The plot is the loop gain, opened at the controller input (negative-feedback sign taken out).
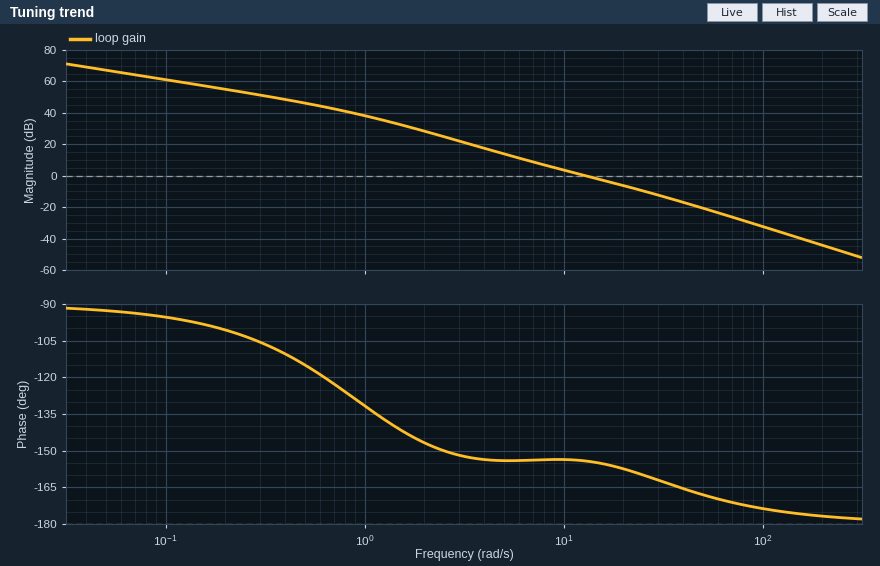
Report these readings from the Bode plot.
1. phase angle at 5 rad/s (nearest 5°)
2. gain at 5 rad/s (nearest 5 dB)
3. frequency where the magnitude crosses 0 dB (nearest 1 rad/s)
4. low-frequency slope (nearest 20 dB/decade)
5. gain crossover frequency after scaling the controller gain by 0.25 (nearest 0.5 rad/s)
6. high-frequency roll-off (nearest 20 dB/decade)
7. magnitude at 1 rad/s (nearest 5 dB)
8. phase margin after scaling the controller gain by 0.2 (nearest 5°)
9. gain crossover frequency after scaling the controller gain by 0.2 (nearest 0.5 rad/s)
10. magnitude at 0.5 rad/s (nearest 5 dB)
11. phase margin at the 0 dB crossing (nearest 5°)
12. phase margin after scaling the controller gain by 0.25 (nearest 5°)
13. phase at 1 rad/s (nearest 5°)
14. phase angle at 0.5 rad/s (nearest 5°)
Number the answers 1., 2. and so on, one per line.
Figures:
1. -155°
2. 15 dB
3. 13 rad/s
4. -20 dB/decade
5. 5.5 rad/s
6. -40 dB/decade
7. 40 dB
8. 25°
9. 5.0 rad/s
10. 45 dB
11. 25°
12. 25°
13. -130°
14. -115°
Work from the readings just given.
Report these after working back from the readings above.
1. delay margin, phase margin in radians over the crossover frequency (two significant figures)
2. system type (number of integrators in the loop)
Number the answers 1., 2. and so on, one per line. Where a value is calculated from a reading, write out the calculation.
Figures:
1. 25 × π / 180 / 13 = 0.034 s
2. 1
